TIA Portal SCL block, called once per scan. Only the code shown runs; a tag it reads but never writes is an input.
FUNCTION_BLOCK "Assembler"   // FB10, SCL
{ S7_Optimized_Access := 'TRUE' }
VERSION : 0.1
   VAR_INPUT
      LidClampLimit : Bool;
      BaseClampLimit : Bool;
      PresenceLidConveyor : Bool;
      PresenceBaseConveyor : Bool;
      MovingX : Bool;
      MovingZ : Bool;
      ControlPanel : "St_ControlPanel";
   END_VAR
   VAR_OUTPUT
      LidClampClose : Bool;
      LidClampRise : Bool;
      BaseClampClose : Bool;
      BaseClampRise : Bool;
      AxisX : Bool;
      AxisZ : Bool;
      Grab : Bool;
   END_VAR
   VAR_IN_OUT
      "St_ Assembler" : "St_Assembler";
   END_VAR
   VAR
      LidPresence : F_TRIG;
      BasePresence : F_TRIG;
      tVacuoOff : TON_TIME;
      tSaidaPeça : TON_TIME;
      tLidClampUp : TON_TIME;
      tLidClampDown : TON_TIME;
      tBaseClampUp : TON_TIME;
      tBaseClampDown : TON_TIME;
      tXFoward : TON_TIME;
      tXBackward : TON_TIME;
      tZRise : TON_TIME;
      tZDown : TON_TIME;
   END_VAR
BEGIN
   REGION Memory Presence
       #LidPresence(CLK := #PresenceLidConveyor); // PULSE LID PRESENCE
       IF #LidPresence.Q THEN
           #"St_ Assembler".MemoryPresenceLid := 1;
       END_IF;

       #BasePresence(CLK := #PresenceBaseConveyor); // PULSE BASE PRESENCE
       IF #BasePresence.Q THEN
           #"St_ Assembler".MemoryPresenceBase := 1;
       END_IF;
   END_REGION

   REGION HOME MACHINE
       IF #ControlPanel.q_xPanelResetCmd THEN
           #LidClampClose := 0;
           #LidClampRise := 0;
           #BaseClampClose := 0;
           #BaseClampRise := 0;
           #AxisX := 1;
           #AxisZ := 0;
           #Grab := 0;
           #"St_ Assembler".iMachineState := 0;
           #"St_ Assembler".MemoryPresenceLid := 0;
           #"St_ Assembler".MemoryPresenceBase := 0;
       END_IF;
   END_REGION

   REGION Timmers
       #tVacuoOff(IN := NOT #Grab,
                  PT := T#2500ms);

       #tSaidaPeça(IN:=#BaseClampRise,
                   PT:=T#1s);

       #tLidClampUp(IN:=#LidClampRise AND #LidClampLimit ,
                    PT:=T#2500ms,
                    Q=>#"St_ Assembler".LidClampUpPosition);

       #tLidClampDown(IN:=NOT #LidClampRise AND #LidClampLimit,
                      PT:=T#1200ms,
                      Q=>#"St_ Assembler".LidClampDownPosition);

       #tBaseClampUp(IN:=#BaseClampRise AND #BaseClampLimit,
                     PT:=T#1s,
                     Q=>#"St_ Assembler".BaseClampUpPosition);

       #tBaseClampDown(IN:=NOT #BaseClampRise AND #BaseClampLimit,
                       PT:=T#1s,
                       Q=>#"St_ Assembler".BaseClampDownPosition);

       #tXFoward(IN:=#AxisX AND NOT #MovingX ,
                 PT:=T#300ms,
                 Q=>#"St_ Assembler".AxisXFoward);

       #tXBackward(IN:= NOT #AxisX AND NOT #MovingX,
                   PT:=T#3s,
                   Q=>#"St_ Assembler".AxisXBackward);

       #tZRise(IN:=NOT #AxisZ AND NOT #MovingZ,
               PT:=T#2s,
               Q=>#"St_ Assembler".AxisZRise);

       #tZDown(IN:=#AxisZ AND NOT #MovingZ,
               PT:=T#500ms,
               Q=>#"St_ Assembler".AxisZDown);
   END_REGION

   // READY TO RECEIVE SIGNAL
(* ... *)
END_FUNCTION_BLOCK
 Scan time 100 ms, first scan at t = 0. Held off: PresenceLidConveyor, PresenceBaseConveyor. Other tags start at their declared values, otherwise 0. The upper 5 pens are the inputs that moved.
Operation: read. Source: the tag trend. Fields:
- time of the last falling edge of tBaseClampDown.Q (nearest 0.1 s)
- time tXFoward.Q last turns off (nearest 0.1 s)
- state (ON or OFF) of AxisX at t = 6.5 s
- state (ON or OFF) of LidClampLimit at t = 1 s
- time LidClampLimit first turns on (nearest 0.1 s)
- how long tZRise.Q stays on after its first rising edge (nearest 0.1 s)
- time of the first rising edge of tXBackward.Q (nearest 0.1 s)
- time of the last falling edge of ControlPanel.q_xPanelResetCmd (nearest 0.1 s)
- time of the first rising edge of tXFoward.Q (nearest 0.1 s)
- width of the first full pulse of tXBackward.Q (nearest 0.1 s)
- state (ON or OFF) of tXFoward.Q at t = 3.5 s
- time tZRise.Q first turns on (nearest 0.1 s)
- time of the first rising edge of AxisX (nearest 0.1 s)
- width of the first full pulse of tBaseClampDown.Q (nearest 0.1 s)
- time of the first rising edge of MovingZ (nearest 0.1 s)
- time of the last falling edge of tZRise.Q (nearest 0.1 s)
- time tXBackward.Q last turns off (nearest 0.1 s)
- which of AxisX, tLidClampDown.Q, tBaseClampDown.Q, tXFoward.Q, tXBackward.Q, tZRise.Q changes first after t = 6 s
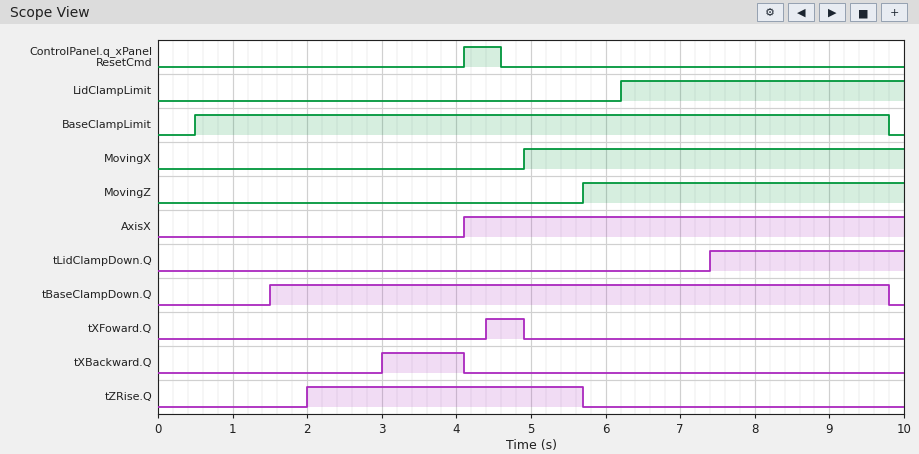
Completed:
9.8 s
4.9 s
ON
OFF
6.2 s
3.7 s
3.0 s
4.6 s
4.4 s
1.1 s
OFF
2.0 s
4.1 s
8.3 s
5.7 s
5.7 s
4.1 s
tLidClampDown.Q
